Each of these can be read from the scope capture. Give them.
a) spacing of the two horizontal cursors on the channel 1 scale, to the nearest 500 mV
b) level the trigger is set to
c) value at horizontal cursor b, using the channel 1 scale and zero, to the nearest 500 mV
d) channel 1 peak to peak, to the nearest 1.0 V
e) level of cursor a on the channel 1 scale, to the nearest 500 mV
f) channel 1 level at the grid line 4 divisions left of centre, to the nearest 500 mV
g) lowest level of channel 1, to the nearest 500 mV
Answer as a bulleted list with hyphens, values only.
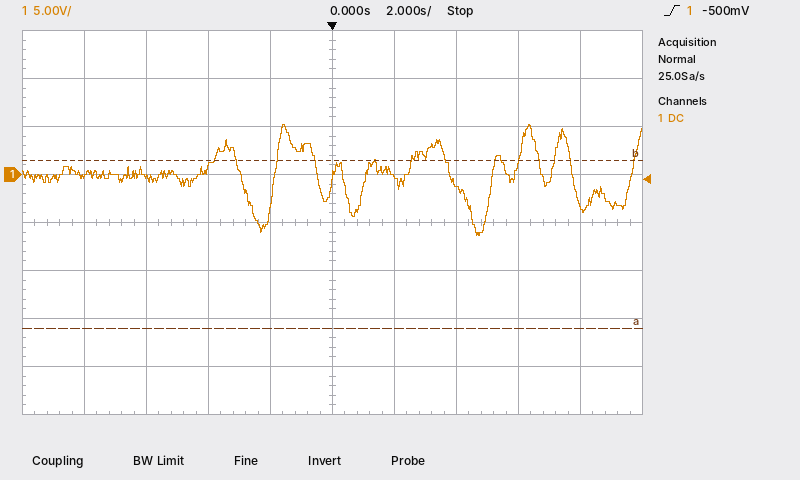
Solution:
- 17.5 V
- -500 mV
- 1.5 V
- 12.0 V
- -16.0 V
- 0.0 V
- -6.5 V
